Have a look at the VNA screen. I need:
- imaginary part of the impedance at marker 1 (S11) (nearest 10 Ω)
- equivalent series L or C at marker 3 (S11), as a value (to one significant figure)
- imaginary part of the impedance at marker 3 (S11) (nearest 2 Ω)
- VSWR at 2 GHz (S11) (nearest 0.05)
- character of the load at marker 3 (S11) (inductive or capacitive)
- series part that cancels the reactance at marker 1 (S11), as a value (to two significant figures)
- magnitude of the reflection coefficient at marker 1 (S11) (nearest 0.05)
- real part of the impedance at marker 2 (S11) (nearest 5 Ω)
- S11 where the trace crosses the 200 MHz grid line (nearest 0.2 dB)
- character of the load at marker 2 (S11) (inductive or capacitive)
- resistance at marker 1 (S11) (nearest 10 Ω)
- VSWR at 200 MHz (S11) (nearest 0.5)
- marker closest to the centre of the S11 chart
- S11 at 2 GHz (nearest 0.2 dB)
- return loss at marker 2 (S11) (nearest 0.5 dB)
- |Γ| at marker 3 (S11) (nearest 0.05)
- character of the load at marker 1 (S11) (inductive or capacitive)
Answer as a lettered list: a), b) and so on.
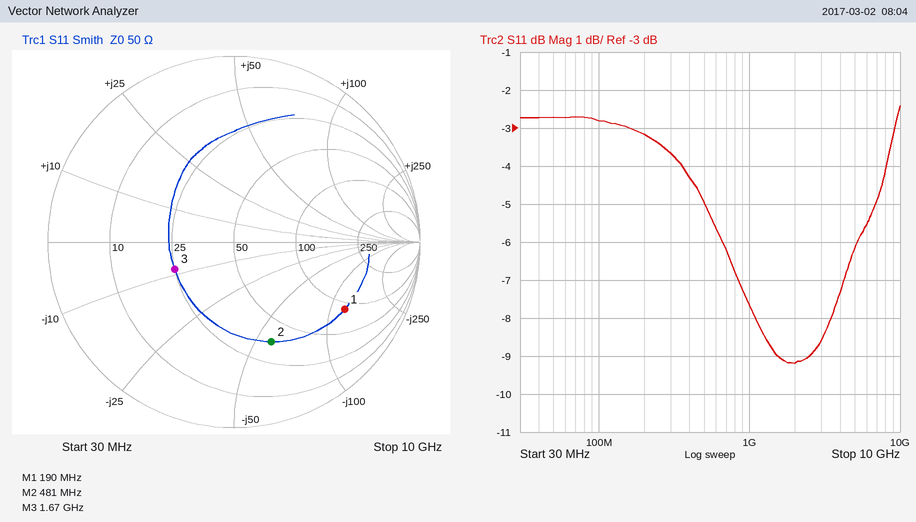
a) -120 Ω
b) 10 pF
c) -8 Ω
d) 2.05
e) capacitive
f) 100 nH
g) 0.70
h) 35 Ω
i) -3.2 dB
j) capacitive
k) 90 Ω
l) 5.5
m) marker 3
n) -9.2 dB
o) 5.0 dB
p) 0.35
q) capacitive
